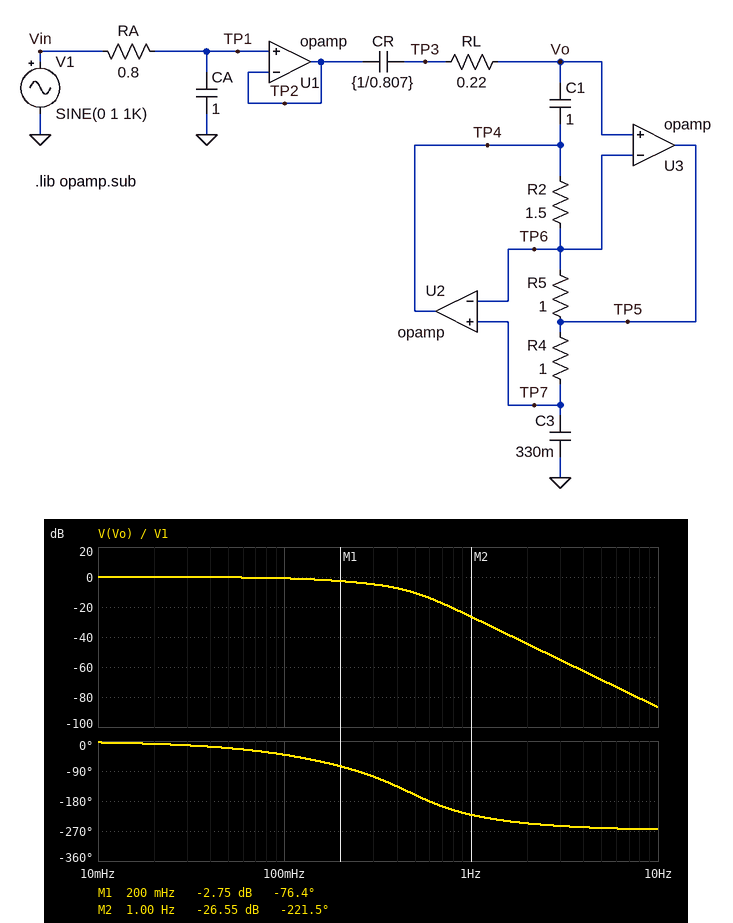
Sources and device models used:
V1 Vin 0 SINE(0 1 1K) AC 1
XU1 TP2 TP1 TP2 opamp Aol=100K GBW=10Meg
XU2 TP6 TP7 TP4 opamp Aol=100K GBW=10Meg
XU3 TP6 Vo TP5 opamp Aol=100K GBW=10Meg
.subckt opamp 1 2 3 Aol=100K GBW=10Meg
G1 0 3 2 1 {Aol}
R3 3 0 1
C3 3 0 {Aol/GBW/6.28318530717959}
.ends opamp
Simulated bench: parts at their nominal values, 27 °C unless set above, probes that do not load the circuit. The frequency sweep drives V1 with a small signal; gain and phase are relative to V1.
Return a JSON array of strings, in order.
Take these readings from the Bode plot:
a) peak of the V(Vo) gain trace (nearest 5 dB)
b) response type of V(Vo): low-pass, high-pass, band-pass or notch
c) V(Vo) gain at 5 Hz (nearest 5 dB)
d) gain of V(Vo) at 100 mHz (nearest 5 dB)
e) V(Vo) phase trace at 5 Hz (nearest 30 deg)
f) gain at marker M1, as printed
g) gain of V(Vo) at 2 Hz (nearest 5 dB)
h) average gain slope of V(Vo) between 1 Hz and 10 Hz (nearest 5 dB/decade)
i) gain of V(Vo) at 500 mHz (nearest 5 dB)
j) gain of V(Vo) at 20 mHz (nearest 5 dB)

["0 dB", "low-pass", "-70 dB", "0 dB", "-270 deg", "-2.75 dB", "-45 dB", "-60 dB/decade", "-10 dB", "0 dB"]
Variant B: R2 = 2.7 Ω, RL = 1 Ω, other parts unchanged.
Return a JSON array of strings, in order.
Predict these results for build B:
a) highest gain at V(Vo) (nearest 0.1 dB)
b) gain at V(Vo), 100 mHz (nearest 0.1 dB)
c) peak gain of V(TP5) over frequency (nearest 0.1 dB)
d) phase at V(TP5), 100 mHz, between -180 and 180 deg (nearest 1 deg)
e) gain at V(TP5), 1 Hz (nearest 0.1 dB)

["1.4 dB", "1.1 dB", "1.7 dB", "-50 deg", "-37.7 dB"]
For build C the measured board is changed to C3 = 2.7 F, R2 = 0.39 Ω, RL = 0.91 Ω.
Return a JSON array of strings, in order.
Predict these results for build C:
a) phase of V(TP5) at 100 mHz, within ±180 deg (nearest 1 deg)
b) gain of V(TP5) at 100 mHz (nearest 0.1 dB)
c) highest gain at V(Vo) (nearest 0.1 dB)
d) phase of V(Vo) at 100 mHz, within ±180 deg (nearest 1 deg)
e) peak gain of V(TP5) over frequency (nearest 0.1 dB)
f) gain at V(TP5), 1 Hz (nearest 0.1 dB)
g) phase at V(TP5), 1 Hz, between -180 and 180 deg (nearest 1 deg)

["-8 deg", "6.6 dB", "0.8 dB", "-67 deg", "8.6 dB", "-21.0 dB", "-164 deg"]
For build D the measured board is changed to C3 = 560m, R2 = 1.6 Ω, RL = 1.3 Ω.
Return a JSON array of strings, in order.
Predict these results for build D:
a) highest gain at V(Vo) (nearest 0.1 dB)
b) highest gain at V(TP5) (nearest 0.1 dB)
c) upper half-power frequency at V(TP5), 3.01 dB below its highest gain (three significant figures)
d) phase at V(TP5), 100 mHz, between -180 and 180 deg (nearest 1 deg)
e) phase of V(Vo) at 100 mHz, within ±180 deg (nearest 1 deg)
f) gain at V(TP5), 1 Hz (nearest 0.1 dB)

["2.5 dB", "3.3 dB", "172 mHz", "-47 deg", "-67 deg", "-36.0 dB"]
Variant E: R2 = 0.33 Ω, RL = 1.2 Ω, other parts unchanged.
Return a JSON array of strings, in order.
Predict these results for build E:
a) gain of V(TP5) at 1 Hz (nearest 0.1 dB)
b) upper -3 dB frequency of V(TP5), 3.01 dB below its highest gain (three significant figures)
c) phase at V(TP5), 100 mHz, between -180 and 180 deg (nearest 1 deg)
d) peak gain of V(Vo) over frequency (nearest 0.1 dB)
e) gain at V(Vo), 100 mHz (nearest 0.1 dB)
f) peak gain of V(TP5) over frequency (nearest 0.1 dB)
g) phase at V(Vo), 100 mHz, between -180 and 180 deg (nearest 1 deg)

["-19.4 dB", "481 mHz", "-18 deg", "4.8 dB", "-0.5 dB", "7.3 dB", "-30 deg"]
